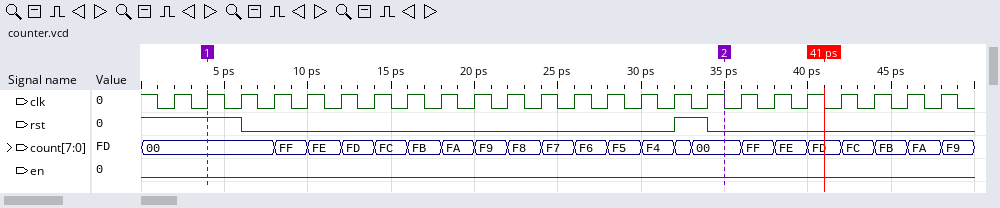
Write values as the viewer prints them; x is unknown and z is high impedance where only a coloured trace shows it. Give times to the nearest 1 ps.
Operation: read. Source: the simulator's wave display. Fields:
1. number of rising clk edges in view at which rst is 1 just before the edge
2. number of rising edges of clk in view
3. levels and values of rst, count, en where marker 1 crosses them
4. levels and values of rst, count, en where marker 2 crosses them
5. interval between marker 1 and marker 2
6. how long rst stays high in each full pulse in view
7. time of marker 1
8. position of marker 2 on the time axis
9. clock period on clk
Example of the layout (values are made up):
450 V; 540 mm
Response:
4; 24; rst=1, count=00, en=0; rst=0, count=00, en=0; 31 ps; 2 ps; 4 ps; 35 ps; 2 ps
